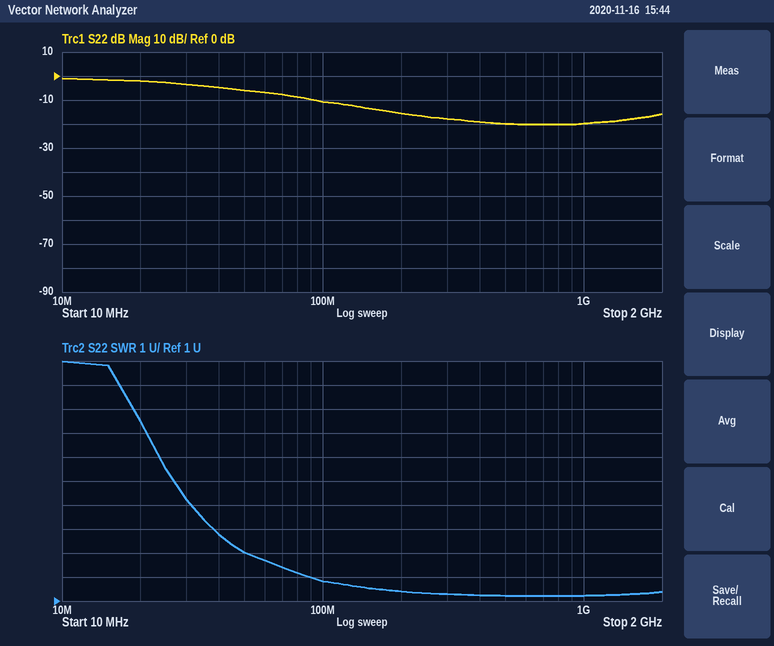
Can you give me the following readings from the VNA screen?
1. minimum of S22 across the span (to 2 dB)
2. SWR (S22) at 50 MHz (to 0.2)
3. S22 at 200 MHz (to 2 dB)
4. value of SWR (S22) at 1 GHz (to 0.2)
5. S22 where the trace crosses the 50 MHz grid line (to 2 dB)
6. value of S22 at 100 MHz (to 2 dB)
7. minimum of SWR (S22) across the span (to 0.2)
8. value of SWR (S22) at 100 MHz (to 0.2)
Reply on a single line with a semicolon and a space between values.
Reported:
-20 dB; 3.0; -16 dB; 1.2; -6 dB; -10 dB; 1.2; 1.8
